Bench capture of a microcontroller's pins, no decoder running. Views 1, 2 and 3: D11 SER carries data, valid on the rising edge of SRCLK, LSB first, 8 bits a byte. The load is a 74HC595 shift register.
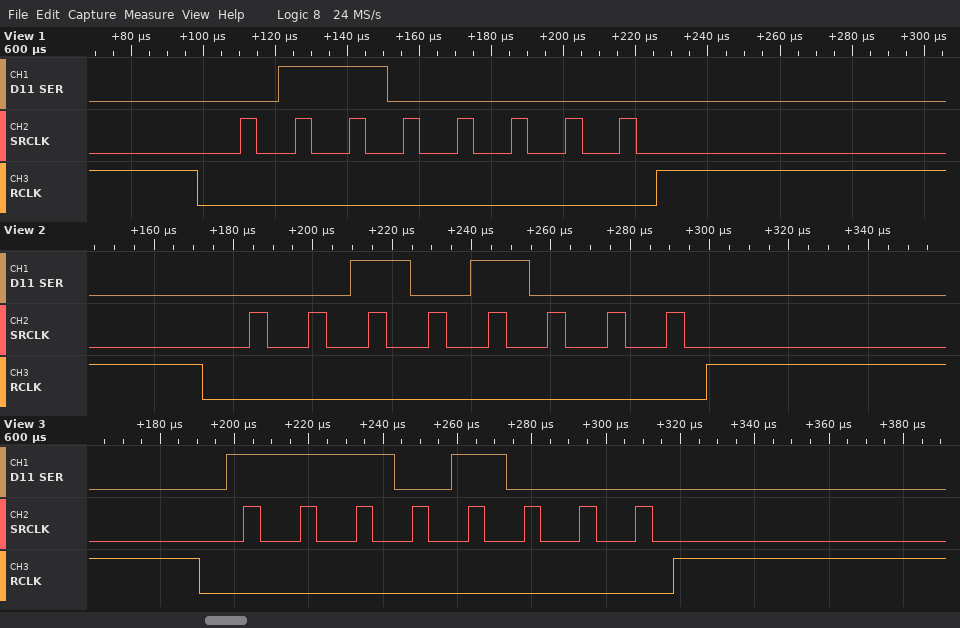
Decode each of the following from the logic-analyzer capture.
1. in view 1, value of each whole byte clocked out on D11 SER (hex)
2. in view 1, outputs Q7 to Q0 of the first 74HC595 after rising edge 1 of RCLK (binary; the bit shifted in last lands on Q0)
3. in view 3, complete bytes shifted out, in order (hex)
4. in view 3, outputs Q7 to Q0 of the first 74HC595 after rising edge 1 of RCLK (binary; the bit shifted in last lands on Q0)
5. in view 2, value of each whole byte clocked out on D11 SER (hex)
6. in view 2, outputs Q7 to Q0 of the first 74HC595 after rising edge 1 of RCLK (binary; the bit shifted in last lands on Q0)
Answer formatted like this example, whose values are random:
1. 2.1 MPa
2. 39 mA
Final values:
1. 06
2. 01100000
3. 0x17
4. 11101000
5. 14
6. 00101000
